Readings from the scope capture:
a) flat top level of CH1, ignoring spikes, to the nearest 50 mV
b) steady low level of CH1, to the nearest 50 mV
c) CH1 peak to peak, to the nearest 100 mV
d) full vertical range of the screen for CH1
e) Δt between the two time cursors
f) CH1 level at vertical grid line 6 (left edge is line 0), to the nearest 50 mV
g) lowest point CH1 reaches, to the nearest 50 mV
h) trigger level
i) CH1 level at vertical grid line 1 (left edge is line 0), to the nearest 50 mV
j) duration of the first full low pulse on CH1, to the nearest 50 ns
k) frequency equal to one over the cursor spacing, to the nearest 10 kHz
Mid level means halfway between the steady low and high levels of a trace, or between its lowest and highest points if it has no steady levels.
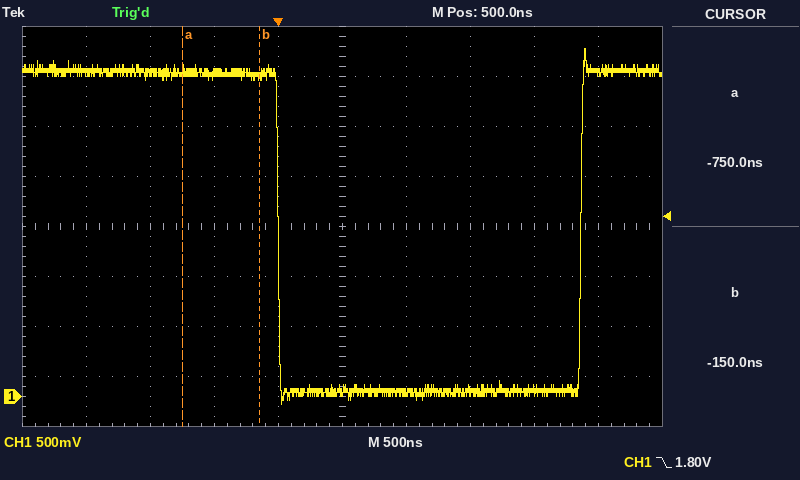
3.25 V
50 mV
3.60 V
4 V
600 ns
50 mV
-100 mV
1.80 V
3.25 V
2.35 µs
1.67 MHz
